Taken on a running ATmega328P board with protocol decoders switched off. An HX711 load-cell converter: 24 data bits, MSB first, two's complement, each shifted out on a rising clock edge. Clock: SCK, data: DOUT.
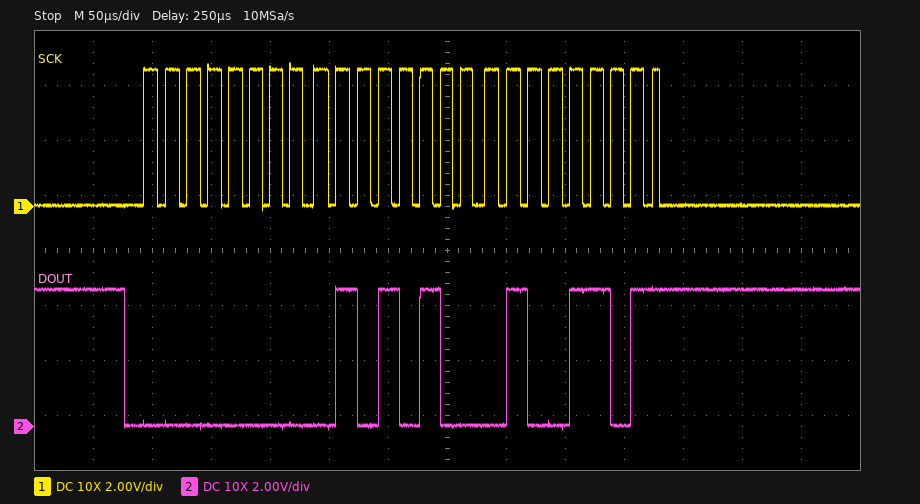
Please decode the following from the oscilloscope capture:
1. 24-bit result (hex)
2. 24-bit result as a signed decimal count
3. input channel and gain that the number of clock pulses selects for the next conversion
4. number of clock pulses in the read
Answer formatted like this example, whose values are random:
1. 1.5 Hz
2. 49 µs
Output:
1. 0x00544D
2. 21581
3. channel A, gain 128
4. 25
